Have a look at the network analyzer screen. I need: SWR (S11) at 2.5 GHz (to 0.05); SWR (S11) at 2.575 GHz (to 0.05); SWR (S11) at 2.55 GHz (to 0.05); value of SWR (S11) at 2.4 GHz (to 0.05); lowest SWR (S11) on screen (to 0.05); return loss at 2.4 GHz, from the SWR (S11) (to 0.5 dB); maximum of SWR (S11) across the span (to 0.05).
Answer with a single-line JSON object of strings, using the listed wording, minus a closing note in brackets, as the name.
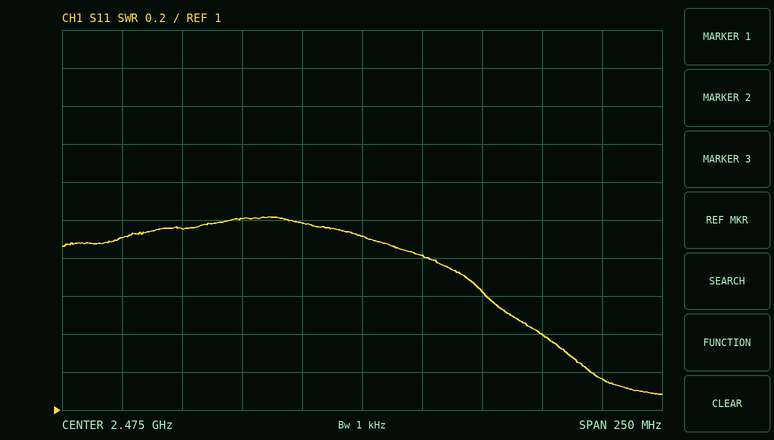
{"SWR (S11) at 2.5 GHz": "1.80", "SWR (S11) at 2.575 GHz": "1.15", "SWR (S11) at 2.55 GHz": "1.40", "value of SWR (S11) at 2.4 GHz": "1.95", "lowest SWR (S11) on screen": "1.10", "return loss at 2.4 GHz, from the SWR (S11)": "10.0 dB", "maximum of SWR (S11) across the span": "2.00"}
